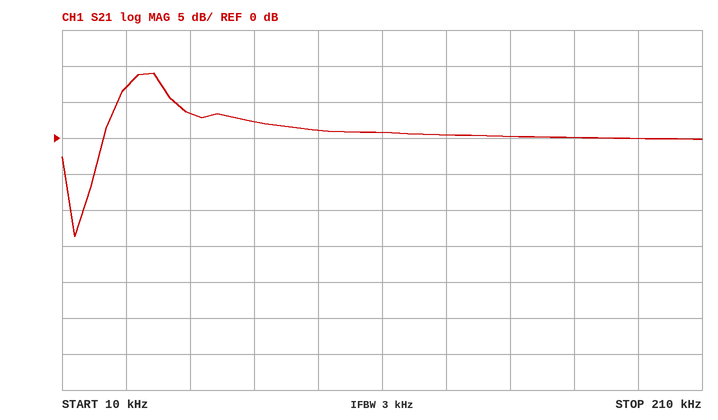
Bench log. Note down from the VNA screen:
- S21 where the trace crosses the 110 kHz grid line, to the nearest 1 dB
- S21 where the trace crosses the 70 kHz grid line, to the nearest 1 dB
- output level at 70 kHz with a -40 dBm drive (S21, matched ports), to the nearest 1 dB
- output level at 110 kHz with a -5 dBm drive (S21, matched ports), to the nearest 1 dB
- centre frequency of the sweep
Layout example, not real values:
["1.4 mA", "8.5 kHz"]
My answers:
["1 dB", "2 dB", "-38 dBm", "-4 dBm", "110 kHz"]
